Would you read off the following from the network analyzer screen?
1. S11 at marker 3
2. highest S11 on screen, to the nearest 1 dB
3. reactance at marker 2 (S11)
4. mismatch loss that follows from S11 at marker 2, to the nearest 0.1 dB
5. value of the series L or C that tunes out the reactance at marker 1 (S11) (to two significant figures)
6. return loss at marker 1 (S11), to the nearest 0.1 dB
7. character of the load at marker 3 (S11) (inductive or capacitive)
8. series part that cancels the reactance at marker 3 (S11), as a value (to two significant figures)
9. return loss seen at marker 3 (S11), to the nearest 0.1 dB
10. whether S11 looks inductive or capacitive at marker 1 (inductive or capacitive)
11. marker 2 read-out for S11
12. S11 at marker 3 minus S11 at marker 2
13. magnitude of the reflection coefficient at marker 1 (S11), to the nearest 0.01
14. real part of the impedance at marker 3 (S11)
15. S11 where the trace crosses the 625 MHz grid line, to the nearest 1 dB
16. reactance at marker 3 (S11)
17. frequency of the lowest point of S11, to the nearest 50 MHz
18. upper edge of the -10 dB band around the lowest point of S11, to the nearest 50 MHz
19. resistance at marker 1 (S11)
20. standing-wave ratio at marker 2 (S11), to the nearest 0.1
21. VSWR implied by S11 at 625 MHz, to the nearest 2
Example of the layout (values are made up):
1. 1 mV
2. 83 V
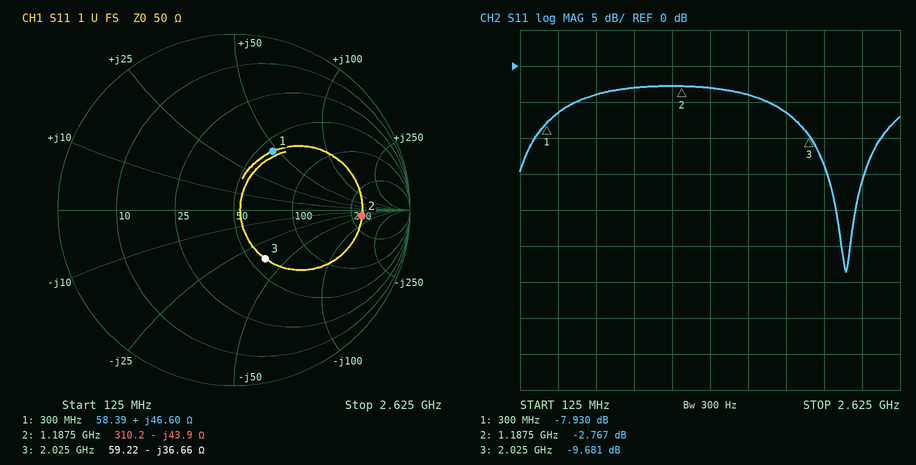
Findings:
1. -9.681 dB
2. -3 dB
3. -43.9 Ω
4. 3.3 dB
5. 11 pF
6. 7.9 dB
7. capacitive
8. 2.9 nH
9. 9.7 dB
10. inductive
11. -2.767 dB
12. -6.914 dB
13. 0.40
14. 59.22 Ω
15. -4 dB
16. -36.66 Ω
17. 2.25 GHz
18. 2.50 GHz
19. 58.39 Ω
20. 6.3
21. 4
